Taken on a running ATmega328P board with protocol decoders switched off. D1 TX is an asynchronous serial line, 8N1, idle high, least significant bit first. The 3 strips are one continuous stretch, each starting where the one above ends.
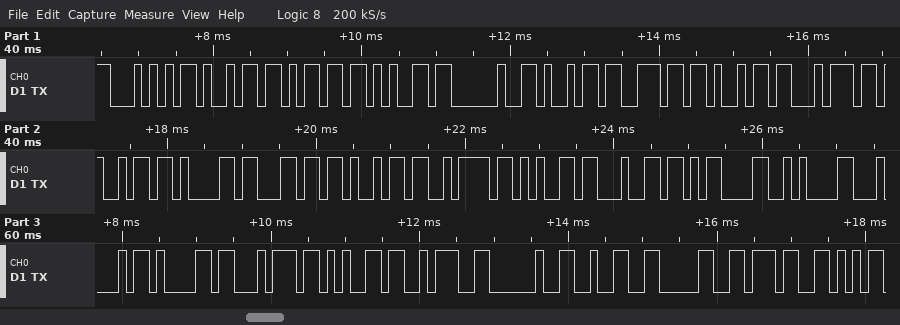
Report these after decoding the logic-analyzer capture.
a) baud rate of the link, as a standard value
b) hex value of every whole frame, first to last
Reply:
9600 baud
0x54 0x69 0x6D 0x65 0x20 0x69 0x6E 0x69 0x74 0x69 0x61 0x6C 0x69 0x7A 0x65 0x64 0x0D 0x0A 0x44 0x61 0x74 0x65 0x3A 0x20 0x32 0x30 0x37
